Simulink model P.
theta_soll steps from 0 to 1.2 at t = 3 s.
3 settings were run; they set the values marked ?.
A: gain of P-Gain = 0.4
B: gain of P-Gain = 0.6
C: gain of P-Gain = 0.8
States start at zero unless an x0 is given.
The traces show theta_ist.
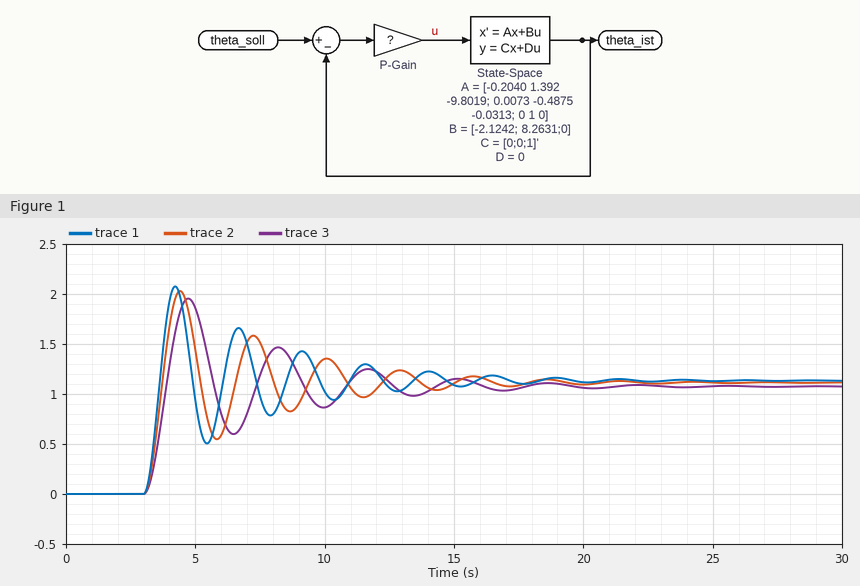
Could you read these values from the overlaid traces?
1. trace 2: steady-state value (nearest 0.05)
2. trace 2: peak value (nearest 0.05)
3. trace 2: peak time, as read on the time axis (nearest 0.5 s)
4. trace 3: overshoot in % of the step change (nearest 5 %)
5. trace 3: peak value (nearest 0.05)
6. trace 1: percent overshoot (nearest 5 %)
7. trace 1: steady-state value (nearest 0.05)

1.10
2.05
4.5 s
80 %
1.95
85 %
1.15
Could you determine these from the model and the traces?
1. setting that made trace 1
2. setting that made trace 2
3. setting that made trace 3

C
B
A
